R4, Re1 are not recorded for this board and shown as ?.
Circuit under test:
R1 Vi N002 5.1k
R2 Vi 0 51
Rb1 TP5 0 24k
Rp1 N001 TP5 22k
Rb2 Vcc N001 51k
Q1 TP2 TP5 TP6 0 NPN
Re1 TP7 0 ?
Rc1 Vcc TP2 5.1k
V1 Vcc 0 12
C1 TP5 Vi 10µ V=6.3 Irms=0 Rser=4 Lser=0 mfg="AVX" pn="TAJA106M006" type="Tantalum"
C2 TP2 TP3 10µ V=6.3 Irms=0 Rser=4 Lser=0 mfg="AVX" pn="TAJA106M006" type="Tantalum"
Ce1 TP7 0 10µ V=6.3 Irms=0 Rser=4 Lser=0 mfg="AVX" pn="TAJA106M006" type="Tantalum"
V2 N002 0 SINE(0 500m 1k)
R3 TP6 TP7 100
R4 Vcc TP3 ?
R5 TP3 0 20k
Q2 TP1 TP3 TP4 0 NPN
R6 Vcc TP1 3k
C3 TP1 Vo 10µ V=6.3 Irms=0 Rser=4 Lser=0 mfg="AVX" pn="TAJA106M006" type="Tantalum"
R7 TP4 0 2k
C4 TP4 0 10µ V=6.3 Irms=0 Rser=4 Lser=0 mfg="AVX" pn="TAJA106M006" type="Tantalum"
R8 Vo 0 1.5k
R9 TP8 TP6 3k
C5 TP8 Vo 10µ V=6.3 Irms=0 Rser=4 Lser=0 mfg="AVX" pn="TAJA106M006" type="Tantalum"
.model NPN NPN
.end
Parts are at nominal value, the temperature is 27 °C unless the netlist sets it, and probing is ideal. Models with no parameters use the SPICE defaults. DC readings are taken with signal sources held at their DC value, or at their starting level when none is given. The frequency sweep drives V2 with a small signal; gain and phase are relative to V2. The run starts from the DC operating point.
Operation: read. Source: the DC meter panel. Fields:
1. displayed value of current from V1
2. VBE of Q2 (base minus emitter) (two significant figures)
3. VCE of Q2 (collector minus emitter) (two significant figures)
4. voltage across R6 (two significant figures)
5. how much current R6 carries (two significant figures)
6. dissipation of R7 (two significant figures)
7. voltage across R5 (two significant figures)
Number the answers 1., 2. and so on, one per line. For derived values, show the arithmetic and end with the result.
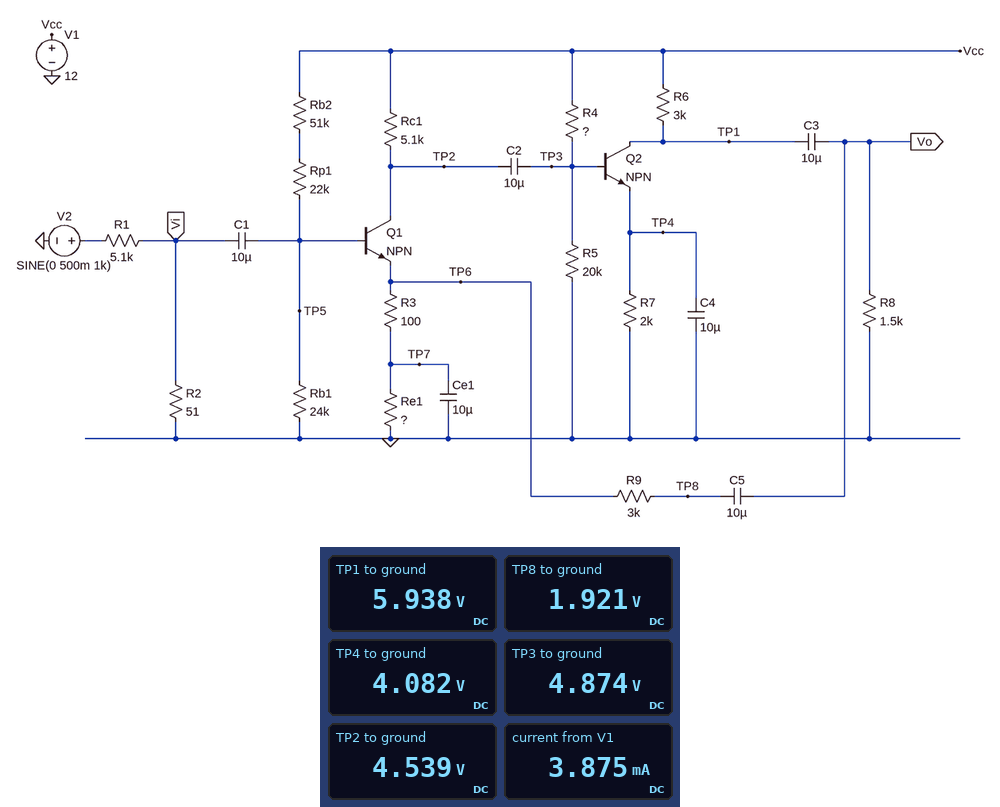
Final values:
1. 3.875 mA
2. 4.874 V - 4.082 V = 790 mV
3. 5.938 V - 4.082 V = 1.9 V
4. 12 V - 5.938 V = 6.1 V
5. (12 V - 5.938 V) / 3 kΩ = 2.0 mA
6. (4.082 V)^2 / 2 kΩ = 8.3 mW
7. 4.874 V = 4.9 V
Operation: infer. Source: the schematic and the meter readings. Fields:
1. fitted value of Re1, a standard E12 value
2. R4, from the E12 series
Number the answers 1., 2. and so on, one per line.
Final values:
1. 1.2 kΩ
2. 27 kΩ
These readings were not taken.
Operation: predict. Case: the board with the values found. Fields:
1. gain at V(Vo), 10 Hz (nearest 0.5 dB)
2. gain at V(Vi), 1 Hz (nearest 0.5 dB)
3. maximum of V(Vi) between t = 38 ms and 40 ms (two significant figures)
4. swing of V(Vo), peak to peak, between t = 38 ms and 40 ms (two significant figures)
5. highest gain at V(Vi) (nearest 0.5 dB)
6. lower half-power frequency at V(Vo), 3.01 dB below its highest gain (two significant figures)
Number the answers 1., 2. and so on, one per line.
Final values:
1. -33.0 dB
2. -40.0 dB
3. 4.9 mV
4. 270 mV
5. -40.0 dB
6. 170 Hz
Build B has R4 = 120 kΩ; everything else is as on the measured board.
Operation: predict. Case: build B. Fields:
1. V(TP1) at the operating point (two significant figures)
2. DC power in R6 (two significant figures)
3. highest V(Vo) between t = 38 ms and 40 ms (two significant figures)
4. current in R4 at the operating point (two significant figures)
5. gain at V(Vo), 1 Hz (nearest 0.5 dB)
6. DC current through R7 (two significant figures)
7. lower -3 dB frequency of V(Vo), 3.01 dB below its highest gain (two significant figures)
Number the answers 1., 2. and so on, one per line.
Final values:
1. 11 V
2. 580 µW
3. 130 mV
4. 86 µA
5. -52.0 dB
6. 440 µA
7. 160 Hz
